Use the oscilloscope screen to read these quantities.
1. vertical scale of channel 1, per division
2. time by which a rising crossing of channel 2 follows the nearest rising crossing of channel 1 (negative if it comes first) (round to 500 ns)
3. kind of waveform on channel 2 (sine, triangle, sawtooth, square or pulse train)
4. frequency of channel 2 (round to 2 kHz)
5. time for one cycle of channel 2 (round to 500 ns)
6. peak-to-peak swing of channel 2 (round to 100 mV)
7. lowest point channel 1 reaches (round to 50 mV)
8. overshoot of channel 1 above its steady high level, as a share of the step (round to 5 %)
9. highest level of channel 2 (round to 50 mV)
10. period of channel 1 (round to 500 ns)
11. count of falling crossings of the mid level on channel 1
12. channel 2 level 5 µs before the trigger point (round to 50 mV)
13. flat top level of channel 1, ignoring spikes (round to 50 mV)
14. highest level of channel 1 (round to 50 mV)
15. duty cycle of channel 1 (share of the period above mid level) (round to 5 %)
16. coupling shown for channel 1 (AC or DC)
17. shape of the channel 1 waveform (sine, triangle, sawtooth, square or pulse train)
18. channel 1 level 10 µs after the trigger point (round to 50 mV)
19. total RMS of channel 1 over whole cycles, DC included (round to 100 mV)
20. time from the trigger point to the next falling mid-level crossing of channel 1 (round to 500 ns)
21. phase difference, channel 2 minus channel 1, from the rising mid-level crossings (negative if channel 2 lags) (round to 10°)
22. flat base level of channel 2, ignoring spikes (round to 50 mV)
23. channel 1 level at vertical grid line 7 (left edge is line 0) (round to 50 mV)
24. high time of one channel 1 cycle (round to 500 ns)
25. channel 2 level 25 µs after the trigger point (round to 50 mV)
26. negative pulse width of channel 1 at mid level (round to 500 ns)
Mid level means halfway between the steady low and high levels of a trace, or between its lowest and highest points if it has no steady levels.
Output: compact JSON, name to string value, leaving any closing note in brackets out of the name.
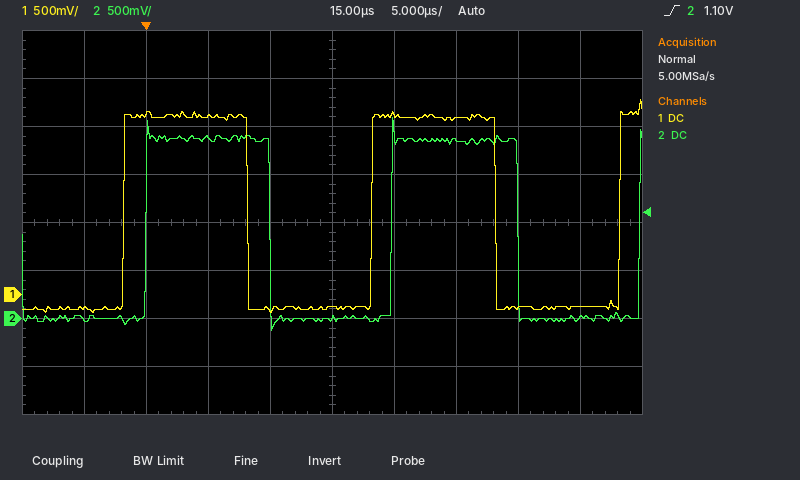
{"vertical scale of channel 1, per division": "500 mV", "time by which a rising crossing of channel 2 follows the nearest rising crossing of channel 1 (negative if it comes first)": "+1.5 µs", "kind of waveform on channel 2": "square", "frequency of channel 2": "50 kHz", "time for one cycle of channel 2": "20.0 µs", "peak-to-peak swing of channel 2": "2.20 V", "lowest point channel 1 reaches": "-200 mV", "overshoot of channel 1 above its steady high level, as a share of the step": "10 %", "highest level of channel 2": "2.10 V", "period of channel 1": "20.0 µs", "count of falling crossings of the mid level on channel 1": "2", "channel 2 level 5 µs before the trigger point": "0 mV", "flat top level of channel 1, ignoring spikes": "1.85 V", "highest level of channel 1": "2.05 V", "duty cycle of channel 1 (share of the period above mid level)": "50 %", "coupling shown for channel 1": "DC", "shape of the channel 1 waveform": "square", "channel 1 level 10 µs after the trigger point": "-150 mV", "total RMS of channel 1 over whole cycles, DC included": "1.3 V", "time from the trigger point to the next falling mid-level crossing of channel 1": "8.0 µs", "phase difference, channel 2 minus channel 1, from the rising mid-level crossings (negative if channel 2 lags)": "-30°", "flat base level of channel 2, ignoring spikes": "0 mV", "channel 1 level at vertical grid line 7 (left edge is line 0)": "1.85 V", "high time of one channel 1 cycle": "10.0 µs", "channel 2 level 25 µs after the trigger point": "1.85 V", "negative pulse width of channel 1 at mid level": "10.0 µs"}
